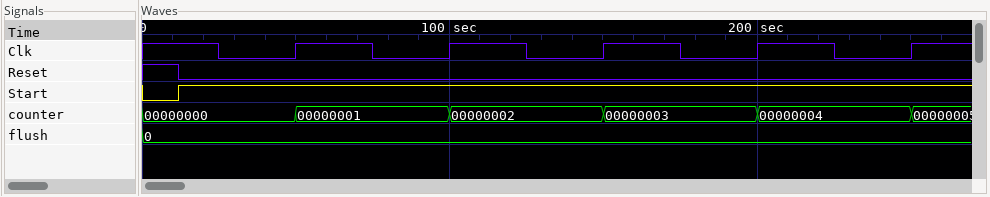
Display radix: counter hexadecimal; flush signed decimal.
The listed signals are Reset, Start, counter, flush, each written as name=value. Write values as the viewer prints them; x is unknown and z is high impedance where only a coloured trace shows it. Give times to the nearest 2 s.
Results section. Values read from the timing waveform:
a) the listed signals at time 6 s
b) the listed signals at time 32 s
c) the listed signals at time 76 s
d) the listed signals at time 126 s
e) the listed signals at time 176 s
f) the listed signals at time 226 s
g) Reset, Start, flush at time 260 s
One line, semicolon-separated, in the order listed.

Reset=1, Start=0, counter=00000000, flush=0; Reset=0, Start=1, counter=00000000, flush=0; Reset=0, Start=1, counter=00000001, flush=0; Reset=0, Start=1, counter=00000002, flush=0; Reset=0, Start=1, counter=00000003, flush=0; Reset=0, Start=1, counter=00000004, flush=0; Reset=0, Start=1, flush=0
